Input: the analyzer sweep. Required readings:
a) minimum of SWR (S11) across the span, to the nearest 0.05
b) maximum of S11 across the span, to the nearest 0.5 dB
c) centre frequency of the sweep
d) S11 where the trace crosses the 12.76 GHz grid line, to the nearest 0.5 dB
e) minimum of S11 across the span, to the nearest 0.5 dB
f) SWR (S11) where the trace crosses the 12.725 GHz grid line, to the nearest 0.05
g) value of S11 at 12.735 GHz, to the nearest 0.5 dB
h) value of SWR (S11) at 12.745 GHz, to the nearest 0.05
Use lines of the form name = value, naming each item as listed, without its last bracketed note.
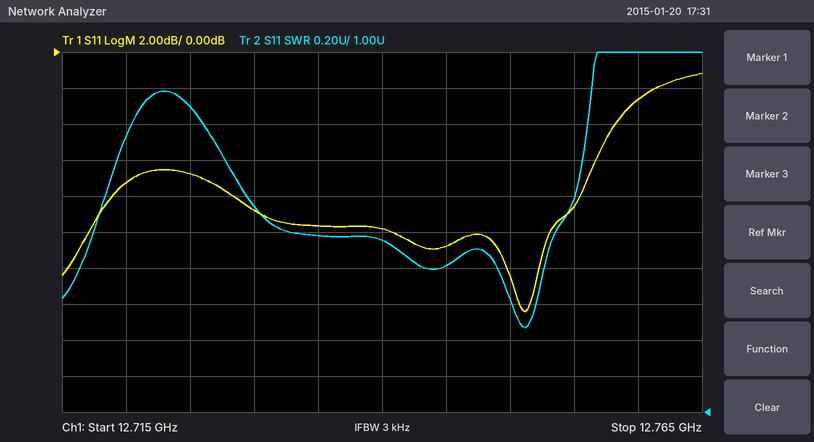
minimum of SWR (S11) across the span, to the nearest 0.05 = 1.45
maximum of S11 across the span, to the nearest 0.5 dB = -1.0 dB
centre frequency of the sweep = 12.74 GHz
S11 where the trace crosses the 12.76 GHz grid line, to the nearest 0.5 dB = -2.5 dB
minimum of S11 across the span, to the nearest 0.5 dB = -14.5 dB
SWR (S11) where the trace crosses the 12.725 GHz grid line, to the nearest 0.05 = 2.70
value of S11 at 12.735 GHz, to the nearest 0.5 dB = -9.5 dB
value of SWR (S11) at 12.745 GHz, to the nearest 0.05 = 1.80
